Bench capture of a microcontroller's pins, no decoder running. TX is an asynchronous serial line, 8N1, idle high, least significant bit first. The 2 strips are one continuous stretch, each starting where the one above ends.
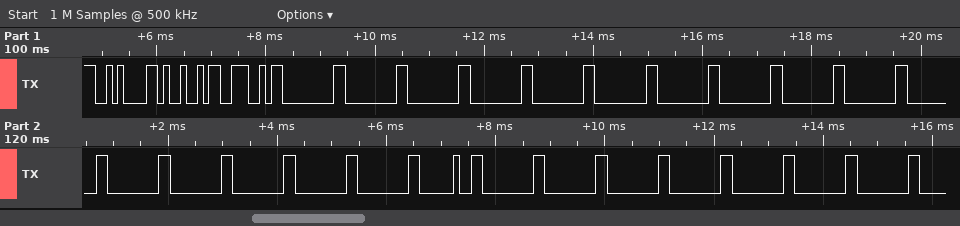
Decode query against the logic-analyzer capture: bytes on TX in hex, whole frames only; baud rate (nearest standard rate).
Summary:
0A 49 4E 00 00 00 00 00 00 00 00 00 00 00 00 00 00 00 00 20 00 00 00 00 00 00 00
9600 baud
